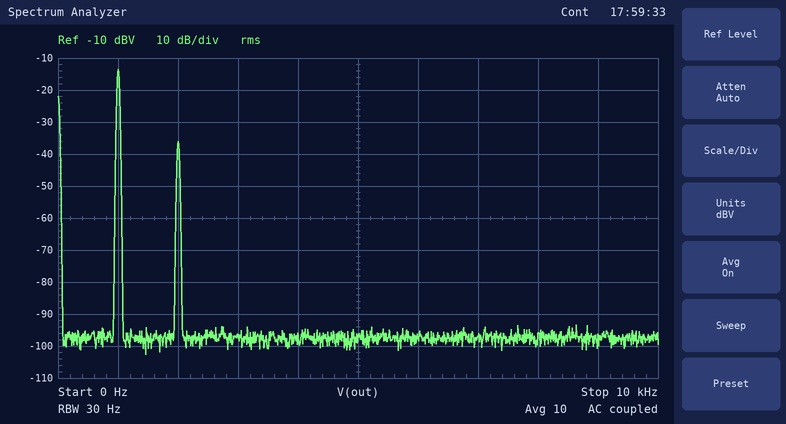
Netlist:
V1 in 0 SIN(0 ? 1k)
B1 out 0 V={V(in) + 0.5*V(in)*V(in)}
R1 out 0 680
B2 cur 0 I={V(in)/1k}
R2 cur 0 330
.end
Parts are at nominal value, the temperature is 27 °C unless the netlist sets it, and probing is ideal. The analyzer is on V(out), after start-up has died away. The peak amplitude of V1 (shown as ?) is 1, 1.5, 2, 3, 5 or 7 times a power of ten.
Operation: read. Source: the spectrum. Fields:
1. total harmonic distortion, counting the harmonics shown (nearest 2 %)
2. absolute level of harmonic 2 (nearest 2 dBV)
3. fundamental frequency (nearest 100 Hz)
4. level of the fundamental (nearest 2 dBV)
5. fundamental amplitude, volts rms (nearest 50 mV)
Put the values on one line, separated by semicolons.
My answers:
8 %; -36 dBV; 1.0 kHz; -14 dBV; 200 mV
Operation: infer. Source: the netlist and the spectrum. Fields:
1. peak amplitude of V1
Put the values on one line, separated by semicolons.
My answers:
300 mV
